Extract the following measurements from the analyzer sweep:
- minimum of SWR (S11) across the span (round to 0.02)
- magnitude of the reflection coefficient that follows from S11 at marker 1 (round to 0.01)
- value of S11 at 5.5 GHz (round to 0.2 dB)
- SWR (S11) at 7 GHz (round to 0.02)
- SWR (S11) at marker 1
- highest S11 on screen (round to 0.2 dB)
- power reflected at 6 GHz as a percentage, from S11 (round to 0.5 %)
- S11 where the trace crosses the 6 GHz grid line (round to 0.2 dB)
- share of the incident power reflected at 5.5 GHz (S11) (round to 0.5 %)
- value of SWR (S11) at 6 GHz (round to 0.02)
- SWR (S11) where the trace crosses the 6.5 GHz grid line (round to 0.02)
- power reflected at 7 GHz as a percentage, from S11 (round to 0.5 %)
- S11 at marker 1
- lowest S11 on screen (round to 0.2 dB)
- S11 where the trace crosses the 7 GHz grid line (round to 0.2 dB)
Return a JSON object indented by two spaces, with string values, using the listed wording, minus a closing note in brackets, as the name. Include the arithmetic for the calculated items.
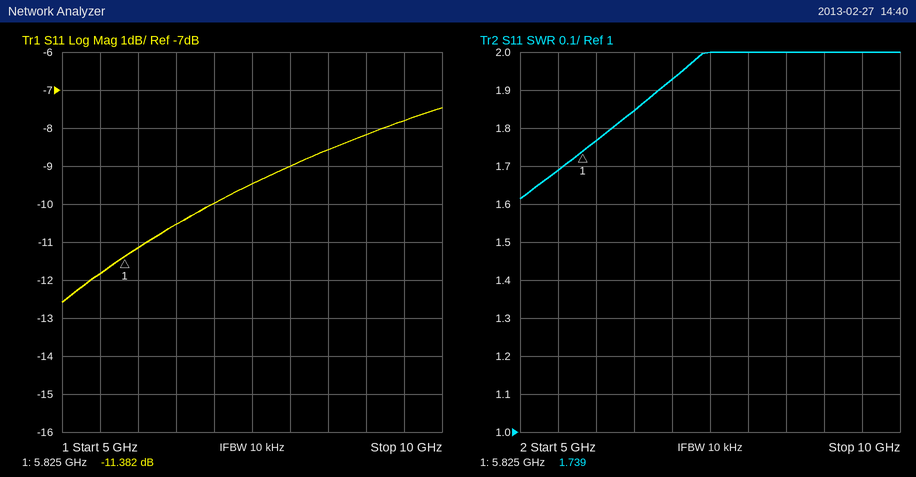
{
  "minimum of SWR (S11) across the span": "1.62",
  "magnitude of the reflection coefficient that follows from S11 at marker 1": "10^(-11.382/20) ≈ 0.27",
  "value of S11 at 5.5 GHz": "-11.8 dB",
  "SWR (S11) at 7 GHz": "1.92",
  "SWR (S11) at marker 1": "1.739",
  "highest S11 on screen": "-7.4 dB",
  "power reflected at 6 GHz as a percentage, from S11": "10^(-11.2/10) ≈ 7.59 %, so 7.5 % to the nearest 0.5 %",
  "S11 where the trace crosses the 6 GHz grid line": "-11.2 dB",
  "share of the incident power reflected at 5.5 GHz (S11)": "10^(-11.8/10) ≈ 6.61 %, so 6.5 % to the nearest 0.5 %",
  "value of SWR (S11) at 6 GHz": "1.76",
  "SWR (S11) where the trace crosses the 6.5 GHz grid line": "1.84",
  "power reflected at 7 GHz as a percentage, from S11": "10^(-10/10) ≈ 10.0 %",
  "S11 at marker 1": "-11.382 dB",
  "lowest S11 on screen": "-12.6 dB",
  "S11 where the trace crosses the 7 GHz grid line": "-10.0 dB"
}
